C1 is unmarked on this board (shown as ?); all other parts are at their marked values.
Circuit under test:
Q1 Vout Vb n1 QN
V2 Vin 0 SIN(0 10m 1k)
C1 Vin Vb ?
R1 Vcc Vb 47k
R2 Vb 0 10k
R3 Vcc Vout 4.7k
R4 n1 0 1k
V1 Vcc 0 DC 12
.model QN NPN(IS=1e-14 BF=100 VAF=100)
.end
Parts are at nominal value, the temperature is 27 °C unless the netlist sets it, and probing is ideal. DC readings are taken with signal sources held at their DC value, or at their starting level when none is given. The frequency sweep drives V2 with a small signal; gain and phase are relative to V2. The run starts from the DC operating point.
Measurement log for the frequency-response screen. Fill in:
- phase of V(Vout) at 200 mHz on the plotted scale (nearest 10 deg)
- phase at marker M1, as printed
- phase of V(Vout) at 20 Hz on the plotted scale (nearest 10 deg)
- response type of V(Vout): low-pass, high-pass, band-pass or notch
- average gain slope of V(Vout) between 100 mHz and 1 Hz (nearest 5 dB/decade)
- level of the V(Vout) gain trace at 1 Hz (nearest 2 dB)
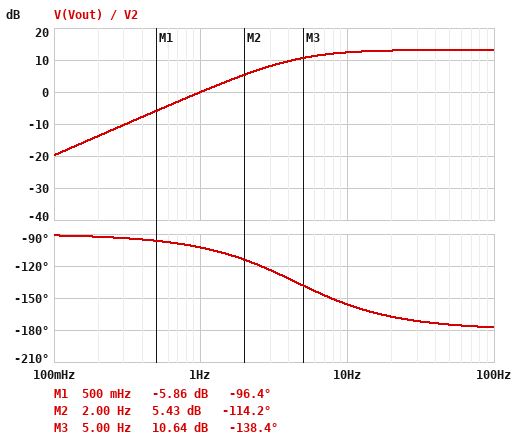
-90 deg
-96.4 deg
-170 deg
high-pass
20 dB/decade
0 dB
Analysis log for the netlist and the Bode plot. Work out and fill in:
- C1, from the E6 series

4.7 µF
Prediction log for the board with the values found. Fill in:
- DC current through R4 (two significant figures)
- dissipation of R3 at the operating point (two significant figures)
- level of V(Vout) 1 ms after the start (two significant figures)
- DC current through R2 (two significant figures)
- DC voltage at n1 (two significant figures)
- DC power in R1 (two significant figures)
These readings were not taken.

1.3 mA
8.3 mW
5.8 V
200 µA
1.3 V
2.1 mW
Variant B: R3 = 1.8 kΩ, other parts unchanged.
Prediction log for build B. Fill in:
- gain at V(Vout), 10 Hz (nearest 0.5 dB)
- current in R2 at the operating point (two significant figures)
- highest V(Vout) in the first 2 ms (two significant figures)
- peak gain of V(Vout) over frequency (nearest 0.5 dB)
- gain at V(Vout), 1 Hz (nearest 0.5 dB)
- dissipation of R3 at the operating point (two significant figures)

4.0 dB
200 µA
9.6 V
5.0 dB
-8.5 dB
3.2 mW
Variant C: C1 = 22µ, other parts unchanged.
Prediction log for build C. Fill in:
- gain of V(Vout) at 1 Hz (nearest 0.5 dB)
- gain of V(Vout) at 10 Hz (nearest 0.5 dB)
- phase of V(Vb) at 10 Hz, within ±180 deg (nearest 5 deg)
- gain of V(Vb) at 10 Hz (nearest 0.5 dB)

10.5 dB
13.0 dB
5 deg
0 dB
